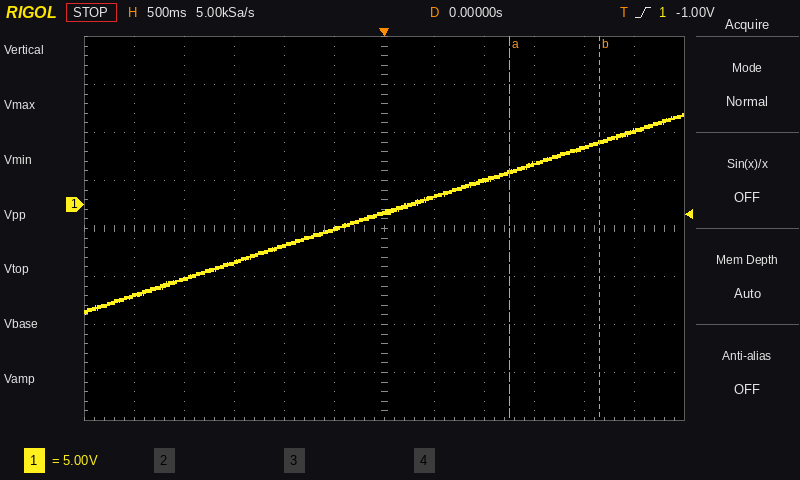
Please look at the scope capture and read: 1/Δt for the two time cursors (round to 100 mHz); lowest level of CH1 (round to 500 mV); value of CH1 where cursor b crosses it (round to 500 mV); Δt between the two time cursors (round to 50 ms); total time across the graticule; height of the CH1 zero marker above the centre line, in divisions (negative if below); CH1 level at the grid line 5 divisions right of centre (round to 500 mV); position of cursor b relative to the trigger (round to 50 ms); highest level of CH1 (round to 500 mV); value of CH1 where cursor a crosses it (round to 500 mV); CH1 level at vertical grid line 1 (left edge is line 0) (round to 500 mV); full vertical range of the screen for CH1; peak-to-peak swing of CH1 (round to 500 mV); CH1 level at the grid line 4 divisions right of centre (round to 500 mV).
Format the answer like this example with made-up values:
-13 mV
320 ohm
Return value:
1.1 Hz
-11.5 V
6.5 V
900 ms
6 s
+0.5 div
7.5 V
+2.15 s
9.5 V
3.5 V
-9.5 V
40 V
21.0 V
6.0 V
